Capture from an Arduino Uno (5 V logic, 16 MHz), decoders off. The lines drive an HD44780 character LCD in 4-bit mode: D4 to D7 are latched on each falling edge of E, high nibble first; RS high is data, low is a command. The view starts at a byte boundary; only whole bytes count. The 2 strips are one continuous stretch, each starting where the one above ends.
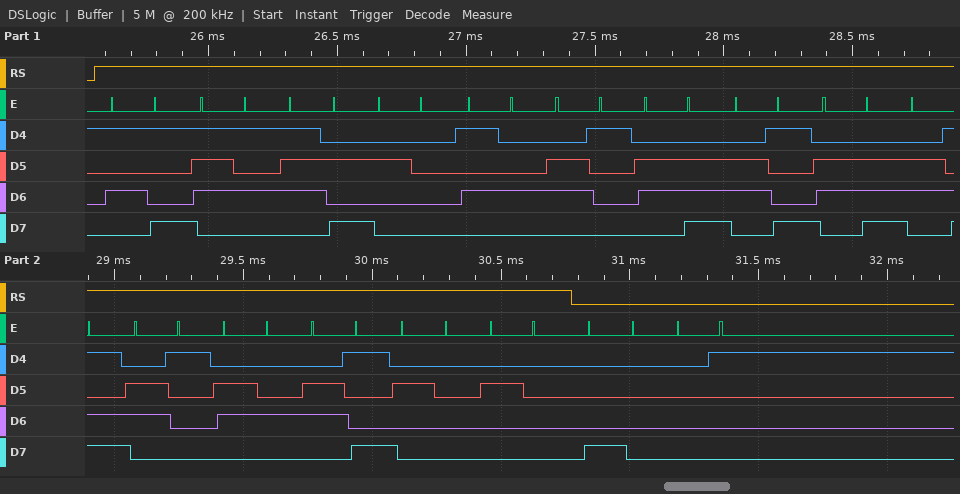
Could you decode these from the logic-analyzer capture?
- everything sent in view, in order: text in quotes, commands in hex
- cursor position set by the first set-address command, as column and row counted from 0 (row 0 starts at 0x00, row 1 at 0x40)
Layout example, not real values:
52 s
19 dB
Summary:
"Yuz Taninmadi  " 0x80 0x01
column 0, row 0
